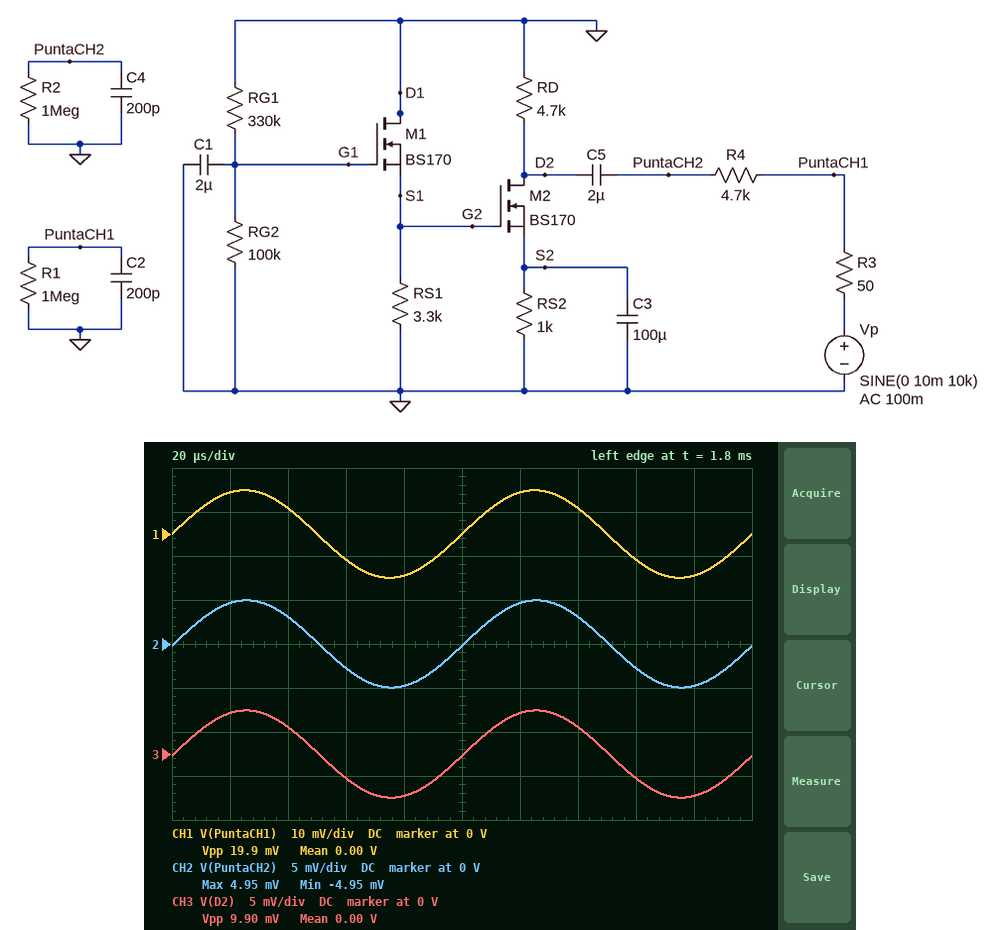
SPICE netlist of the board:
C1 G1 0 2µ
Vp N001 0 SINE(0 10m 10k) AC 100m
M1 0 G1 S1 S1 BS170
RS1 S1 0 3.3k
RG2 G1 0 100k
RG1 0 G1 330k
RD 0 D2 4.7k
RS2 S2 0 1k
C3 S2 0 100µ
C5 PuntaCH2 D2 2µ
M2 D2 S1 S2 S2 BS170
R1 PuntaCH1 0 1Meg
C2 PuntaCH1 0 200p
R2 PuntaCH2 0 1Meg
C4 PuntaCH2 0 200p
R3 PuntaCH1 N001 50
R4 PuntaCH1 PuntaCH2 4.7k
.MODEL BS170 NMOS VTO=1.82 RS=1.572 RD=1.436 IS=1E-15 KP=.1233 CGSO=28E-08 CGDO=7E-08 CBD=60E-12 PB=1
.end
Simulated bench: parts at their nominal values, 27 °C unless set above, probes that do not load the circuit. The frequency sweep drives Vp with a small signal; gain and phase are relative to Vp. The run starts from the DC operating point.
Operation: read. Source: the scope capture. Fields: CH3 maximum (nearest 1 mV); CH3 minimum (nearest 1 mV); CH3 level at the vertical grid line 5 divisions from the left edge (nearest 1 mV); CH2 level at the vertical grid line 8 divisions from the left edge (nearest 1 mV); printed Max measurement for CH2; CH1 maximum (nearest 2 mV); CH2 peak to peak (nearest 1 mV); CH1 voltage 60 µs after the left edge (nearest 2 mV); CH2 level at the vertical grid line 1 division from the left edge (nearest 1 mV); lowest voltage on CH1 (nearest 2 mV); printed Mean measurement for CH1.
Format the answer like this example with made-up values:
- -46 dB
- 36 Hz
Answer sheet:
- 5 mV
- -5 mV
- 0 V
- -3 mV
- 4.95 mV
- 10 mV
- 10 mV
- -6 mV
- 5 mV
- -10 mV
- 0.00 V
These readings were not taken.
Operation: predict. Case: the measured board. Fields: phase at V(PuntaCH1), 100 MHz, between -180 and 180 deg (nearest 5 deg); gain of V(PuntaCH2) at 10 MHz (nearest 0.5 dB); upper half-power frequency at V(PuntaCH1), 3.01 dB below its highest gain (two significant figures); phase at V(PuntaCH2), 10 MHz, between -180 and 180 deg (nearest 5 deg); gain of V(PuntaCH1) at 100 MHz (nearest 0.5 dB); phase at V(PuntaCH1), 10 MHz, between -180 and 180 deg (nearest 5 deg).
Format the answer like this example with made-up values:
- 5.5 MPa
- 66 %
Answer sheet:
- -80 deg
- -39.5 dB
- 16 MHz
- -120 deg
- -16.0 dB
- -30 deg
